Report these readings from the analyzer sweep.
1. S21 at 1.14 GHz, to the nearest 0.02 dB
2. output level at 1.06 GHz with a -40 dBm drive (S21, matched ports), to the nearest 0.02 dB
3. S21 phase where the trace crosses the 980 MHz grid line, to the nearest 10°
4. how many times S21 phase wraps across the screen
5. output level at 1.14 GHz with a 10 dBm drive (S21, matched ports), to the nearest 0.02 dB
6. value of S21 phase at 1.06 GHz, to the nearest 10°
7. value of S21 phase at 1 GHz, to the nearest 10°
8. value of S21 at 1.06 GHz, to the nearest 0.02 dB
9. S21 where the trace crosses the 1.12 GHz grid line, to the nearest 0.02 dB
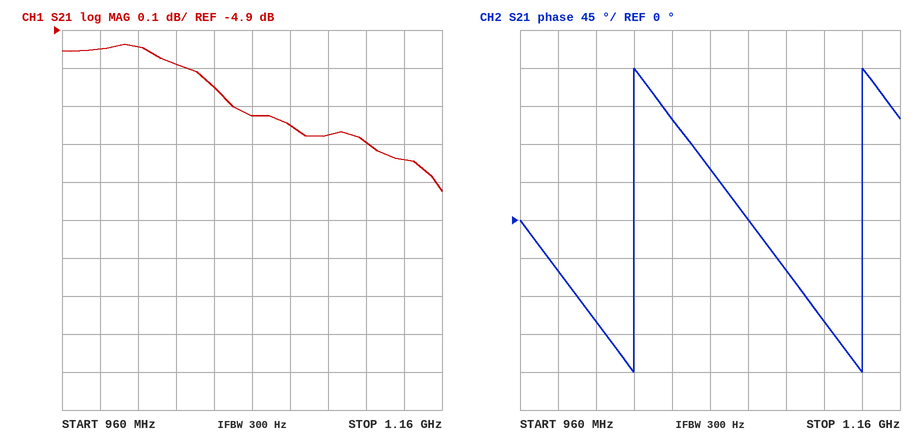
-5.24 dB
-45.12 dBm
-60°
2
4.76 dBm
60°
-120°
-5.12 dB
-5.20 dB
